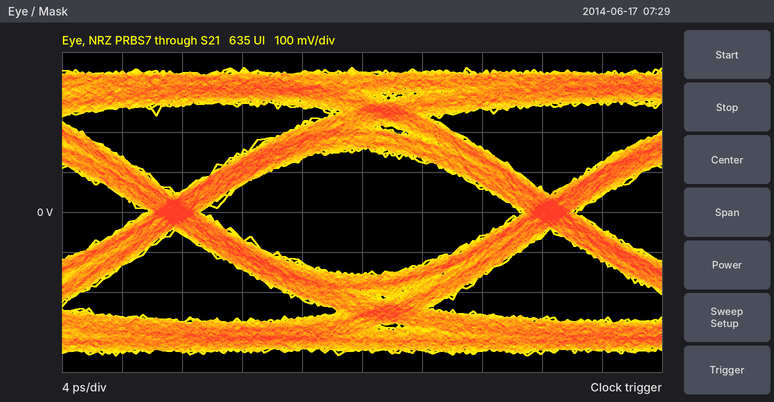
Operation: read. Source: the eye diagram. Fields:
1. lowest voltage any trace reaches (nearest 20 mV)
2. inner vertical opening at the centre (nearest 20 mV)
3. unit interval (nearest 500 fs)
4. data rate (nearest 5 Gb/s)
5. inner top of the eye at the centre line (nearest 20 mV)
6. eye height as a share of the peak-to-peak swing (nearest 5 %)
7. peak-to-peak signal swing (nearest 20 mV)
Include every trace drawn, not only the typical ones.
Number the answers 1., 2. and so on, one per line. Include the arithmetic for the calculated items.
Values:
1. -360 mV
2. 320 mV
3. 25.0 ps
4. 40 Gb/s
5. 160 mV
6. 320 mV / 720 mV ≈ 44.4 %, so 45 % to the nearest 5 %
7. 720 mV
